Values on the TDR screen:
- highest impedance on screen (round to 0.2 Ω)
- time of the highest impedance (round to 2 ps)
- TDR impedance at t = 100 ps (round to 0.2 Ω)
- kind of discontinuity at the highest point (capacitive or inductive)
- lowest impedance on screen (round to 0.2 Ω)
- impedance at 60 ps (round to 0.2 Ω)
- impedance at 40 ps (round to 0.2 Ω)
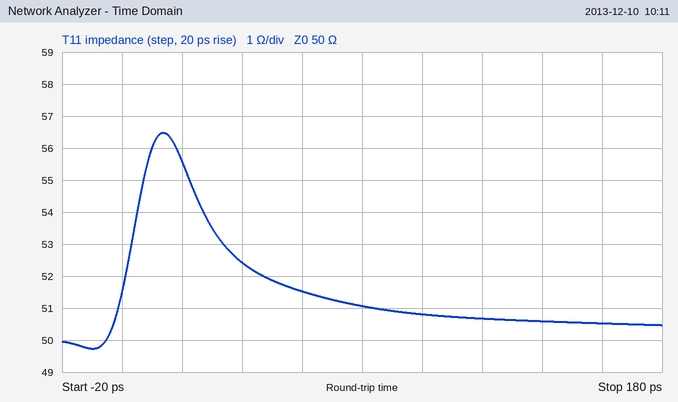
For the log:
56.4 Ω
14 ps
50.8 Ω
inductive
49.8 Ω
51.6 Ω
52.4 Ω
